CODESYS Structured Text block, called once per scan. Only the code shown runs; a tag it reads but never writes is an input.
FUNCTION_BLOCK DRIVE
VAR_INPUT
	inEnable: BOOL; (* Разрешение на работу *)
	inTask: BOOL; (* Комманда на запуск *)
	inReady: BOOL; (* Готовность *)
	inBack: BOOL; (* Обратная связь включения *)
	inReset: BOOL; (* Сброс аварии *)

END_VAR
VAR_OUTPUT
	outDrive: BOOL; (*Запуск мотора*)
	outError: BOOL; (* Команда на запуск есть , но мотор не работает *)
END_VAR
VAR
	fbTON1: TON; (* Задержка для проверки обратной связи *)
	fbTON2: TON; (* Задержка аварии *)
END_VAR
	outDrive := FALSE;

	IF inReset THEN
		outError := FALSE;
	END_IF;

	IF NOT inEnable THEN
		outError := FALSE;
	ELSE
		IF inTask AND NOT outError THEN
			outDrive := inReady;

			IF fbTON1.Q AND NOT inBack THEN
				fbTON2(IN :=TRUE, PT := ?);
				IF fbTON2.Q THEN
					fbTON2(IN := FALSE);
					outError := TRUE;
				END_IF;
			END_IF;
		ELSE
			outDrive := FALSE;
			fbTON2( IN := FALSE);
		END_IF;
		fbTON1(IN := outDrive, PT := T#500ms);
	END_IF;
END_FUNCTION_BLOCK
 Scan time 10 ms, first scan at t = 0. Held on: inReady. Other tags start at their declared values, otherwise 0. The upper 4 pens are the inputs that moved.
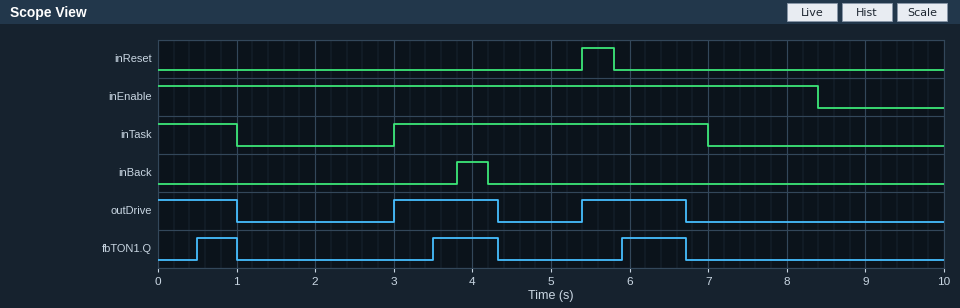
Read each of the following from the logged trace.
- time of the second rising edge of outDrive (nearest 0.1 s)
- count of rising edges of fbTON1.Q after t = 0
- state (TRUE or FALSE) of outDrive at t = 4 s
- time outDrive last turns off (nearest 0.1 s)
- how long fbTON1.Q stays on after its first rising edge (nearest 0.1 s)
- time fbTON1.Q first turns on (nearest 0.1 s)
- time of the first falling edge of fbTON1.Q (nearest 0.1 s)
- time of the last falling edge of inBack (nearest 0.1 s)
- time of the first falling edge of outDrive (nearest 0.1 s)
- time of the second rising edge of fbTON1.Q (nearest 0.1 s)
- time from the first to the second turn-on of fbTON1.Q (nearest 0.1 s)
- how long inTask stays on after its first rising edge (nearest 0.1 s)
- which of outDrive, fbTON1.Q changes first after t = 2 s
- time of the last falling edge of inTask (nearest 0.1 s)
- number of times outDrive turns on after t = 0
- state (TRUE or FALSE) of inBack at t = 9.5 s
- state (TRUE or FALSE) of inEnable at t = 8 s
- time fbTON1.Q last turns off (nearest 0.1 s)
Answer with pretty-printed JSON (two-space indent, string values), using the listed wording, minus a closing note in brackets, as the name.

{
  "time of the second rising edge of outDrive": "5.4 s",
  "count of rising edges of fbTON1.Q after t = 0": "3",
  "state (TRUE or FALSE) of outDrive at t = 4 s": "TRUE",
  "time outDrive last turns off": "6.7 s",
  "how long fbTON1.Q stays on after its first rising edge": "0.5 s",
  "time fbTON1.Q first turns on": "0.5 s",
  "time of the first falling edge of fbTON1.Q": "1.0 s",
  "time of the last falling edge of inBack": "4.2 s",
  "time of the first falling edge of outDrive": "1.0 s",
  "time of the second rising edge of fbTON1.Q": "3.5 s",
  "time from the first to the second turn-on of fbTON1.Q": "3.0 s",
  "how long inTask stays on after its first rising edge": "4.0 s",
  "which of outDrive, fbTON1.Q changes first after t = 2 s": "outDrive",
  "time of the last falling edge of inTask": "7.0 s",
  "number of times outDrive turns on after t = 0": "2",
  "state (TRUE or FALSE) of inBack at t = 9.5 s": "FALSE",
  "state (TRUE or FALSE) of inEnable at t = 8 s": "TRUE",
  "time fbTON1.Q last turns off": "6.7 s"
}
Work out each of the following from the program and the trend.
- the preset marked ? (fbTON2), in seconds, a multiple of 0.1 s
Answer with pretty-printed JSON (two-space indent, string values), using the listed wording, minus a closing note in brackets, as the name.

{
  "the preset marked ? (fbTON2), in seconds, a multiple of 0.1 s": "0.8 s"
}
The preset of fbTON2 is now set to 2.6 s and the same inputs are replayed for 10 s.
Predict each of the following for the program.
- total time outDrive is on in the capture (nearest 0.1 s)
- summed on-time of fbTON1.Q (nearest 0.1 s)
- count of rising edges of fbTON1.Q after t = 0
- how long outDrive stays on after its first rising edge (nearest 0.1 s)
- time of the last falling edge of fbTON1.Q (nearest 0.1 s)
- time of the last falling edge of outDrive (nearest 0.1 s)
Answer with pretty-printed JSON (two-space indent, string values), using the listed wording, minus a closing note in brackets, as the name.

{
  "total time outDrive is on in the capture": "4.1 s",
  "summed on-time of fbTON1.Q": "3.1 s",
  "count of rising edges of fbTON1.Q after t = 0": "2",
  "how long outDrive stays on after its first rising edge": "3.1 s",
  "time of the last falling edge of fbTON1.Q": "6.1 s",
  "time of the last falling edge of outDrive": "6.1 s"
}
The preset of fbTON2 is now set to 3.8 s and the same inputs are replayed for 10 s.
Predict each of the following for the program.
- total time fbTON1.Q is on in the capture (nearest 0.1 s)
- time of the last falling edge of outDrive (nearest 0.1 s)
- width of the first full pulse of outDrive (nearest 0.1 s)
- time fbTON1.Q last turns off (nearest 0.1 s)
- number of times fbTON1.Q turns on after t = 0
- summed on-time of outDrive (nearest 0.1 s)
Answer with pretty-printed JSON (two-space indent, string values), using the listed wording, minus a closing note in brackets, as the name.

{
  "total time fbTON1.Q is on in the capture": "4.0 s",
  "time of the last falling edge of outDrive": "7.0 s",
  "width of the first full pulse of outDrive": "4.0 s",
  "time fbTON1.Q last turns off": "7.0 s",
  "number of times fbTON1.Q turns on after t = 0": "2",
  "summed on-time of outDrive": "5.0 s"
}
